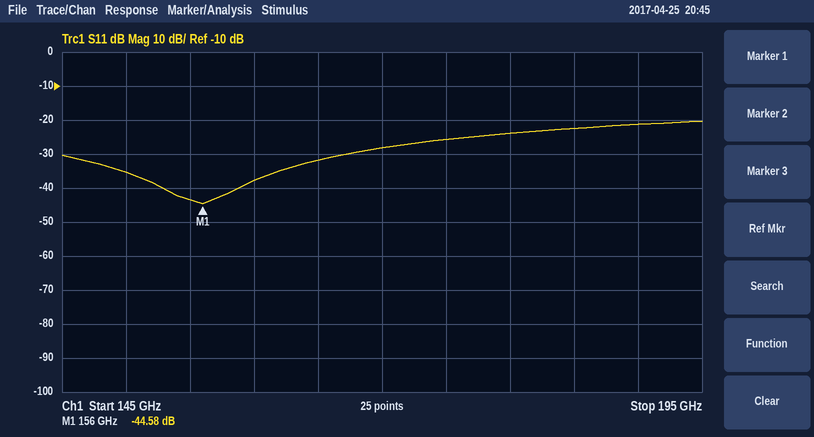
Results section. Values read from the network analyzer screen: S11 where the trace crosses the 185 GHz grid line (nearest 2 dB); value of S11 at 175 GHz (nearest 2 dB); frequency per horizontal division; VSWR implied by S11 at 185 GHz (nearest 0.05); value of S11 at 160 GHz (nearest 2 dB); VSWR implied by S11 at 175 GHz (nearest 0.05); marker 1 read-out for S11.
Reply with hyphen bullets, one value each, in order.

- -22 dB
- -26 dB
- 5 GHz
- 1.15
- -38 dB
- 1.10
- -44.58 dB
